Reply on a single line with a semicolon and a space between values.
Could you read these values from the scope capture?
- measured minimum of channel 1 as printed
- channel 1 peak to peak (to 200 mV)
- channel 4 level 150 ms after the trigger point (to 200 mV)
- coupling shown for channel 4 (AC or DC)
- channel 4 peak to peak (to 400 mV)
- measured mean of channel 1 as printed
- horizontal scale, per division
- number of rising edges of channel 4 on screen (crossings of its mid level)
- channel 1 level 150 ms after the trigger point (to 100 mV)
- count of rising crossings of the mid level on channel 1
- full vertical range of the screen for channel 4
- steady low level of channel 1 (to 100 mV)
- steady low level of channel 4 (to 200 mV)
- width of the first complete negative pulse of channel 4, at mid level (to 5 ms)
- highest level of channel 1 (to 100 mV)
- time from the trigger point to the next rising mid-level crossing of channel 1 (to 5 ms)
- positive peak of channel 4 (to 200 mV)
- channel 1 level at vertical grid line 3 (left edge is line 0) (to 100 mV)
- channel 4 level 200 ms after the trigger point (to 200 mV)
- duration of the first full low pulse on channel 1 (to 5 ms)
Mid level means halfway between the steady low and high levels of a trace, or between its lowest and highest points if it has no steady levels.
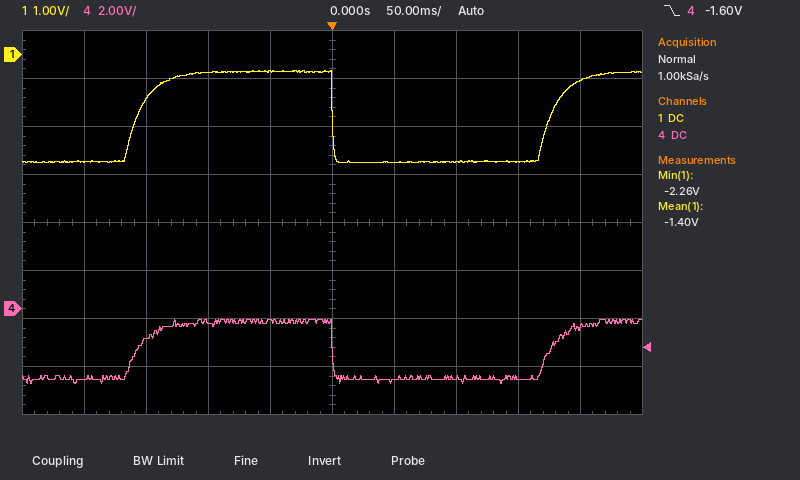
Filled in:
-2.26 V; 2.0 V; -2.8 V; DC; 2.8 V; -1.40 V; 50 ms; 2; -2.2 V; 2; 16 V; -2.2 V; -3.0 V; 175 ms; -300 mV; 175 ms; -400 mV; -400 mV; -800 mV; 175 ms
